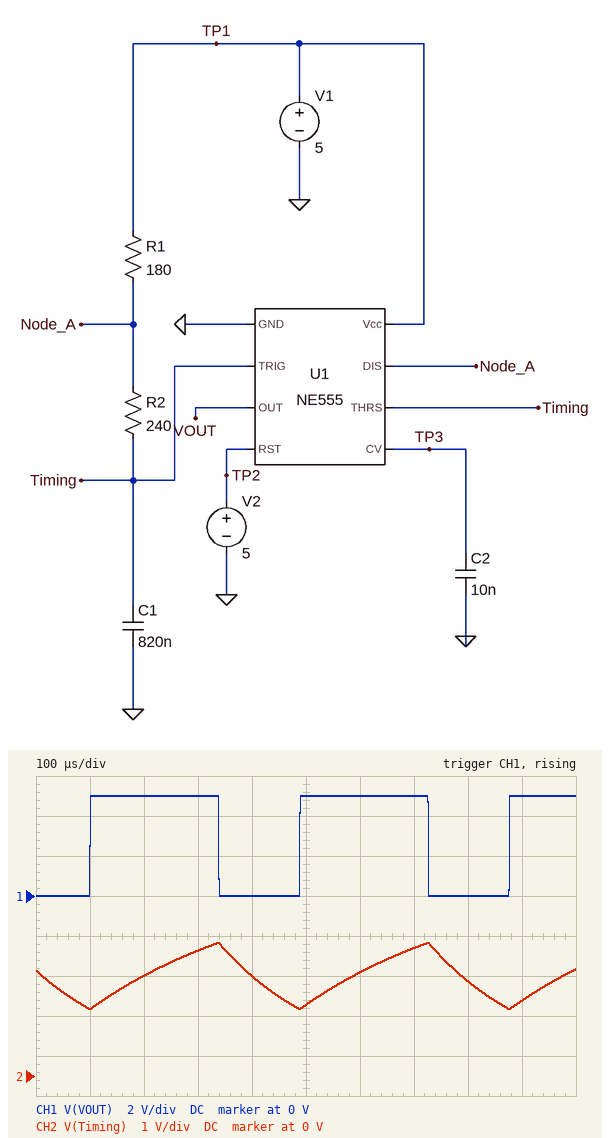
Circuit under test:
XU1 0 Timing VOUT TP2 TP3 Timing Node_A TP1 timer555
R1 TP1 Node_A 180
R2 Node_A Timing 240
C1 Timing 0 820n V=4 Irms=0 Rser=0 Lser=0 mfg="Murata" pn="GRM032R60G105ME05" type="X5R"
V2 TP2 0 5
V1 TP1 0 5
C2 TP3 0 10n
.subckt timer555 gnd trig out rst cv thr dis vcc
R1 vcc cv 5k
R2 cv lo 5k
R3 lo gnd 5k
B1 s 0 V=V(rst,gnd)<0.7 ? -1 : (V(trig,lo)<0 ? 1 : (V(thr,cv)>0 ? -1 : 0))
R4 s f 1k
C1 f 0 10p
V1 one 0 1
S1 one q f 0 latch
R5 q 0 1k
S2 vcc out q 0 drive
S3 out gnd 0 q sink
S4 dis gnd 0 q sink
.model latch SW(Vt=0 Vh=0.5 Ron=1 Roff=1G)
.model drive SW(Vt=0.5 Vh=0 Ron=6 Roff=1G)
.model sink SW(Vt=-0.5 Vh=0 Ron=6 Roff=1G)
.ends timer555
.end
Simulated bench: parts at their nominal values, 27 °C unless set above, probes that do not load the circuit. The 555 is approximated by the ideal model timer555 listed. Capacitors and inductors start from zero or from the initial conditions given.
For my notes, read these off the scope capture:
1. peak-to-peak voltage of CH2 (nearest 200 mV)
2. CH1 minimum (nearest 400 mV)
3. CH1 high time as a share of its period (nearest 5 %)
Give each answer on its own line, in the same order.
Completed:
1.6 V
0 V
60 %
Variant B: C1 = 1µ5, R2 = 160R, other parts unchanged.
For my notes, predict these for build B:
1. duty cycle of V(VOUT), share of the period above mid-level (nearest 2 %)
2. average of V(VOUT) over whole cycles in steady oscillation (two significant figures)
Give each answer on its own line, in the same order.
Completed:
66 %
3.3 V
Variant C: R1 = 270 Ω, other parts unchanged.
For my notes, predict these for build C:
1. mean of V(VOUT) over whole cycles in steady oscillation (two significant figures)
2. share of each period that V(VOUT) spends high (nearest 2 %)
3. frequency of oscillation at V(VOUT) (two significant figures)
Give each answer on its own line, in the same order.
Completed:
3.3 V
66 %
2.3 kHz
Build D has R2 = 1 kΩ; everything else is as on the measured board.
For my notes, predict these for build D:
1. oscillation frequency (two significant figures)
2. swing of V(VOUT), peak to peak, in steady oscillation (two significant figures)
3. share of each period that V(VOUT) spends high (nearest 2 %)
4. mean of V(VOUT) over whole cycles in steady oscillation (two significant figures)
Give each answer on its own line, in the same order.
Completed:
780 Hz
5.0 V
52 %
2.6 V
